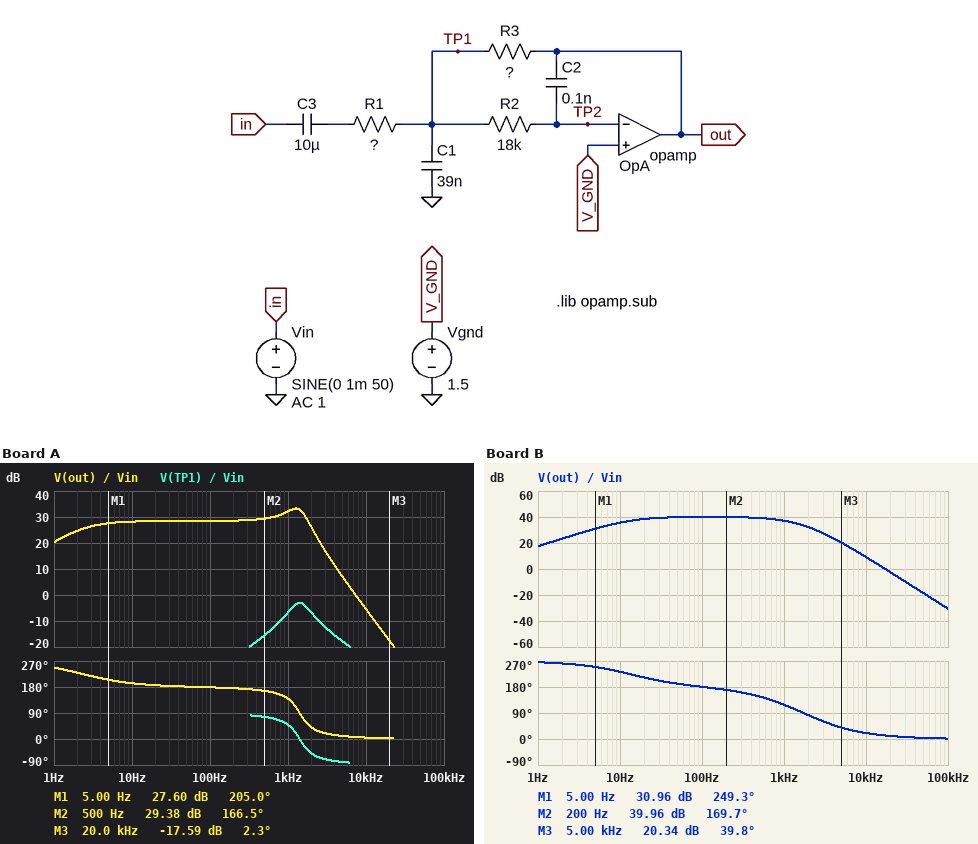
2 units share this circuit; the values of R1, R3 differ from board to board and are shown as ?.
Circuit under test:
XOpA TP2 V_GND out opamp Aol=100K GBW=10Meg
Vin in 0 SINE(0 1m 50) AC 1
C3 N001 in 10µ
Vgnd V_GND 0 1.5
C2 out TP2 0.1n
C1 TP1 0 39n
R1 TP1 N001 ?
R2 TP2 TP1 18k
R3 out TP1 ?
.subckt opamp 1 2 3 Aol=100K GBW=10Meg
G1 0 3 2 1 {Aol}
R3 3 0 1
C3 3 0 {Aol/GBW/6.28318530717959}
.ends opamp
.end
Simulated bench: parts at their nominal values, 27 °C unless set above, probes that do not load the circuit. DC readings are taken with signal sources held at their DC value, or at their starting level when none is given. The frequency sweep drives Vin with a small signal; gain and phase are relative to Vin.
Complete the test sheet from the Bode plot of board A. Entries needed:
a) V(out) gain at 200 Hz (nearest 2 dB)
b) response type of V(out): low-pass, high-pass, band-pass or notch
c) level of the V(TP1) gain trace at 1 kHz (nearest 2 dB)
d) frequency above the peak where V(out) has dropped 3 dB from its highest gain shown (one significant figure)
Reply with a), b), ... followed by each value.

a) 28 dB
b) band-pass
c) -6 dB
d) 2 kHz
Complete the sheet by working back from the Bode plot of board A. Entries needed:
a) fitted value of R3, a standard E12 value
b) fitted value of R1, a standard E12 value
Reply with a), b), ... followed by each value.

a) 180 kΩ
b) 6.8 kΩ
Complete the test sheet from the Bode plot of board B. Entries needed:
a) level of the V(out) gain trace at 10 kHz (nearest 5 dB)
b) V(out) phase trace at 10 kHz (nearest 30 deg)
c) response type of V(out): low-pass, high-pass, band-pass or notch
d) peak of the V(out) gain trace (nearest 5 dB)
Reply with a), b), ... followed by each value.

a) 10 dB
b) 30 deg
c) band-pass
d) 40 dB
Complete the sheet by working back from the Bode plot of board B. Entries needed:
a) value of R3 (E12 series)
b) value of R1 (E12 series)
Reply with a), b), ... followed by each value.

a) 120 kΩ
b) 1.2 kΩ
